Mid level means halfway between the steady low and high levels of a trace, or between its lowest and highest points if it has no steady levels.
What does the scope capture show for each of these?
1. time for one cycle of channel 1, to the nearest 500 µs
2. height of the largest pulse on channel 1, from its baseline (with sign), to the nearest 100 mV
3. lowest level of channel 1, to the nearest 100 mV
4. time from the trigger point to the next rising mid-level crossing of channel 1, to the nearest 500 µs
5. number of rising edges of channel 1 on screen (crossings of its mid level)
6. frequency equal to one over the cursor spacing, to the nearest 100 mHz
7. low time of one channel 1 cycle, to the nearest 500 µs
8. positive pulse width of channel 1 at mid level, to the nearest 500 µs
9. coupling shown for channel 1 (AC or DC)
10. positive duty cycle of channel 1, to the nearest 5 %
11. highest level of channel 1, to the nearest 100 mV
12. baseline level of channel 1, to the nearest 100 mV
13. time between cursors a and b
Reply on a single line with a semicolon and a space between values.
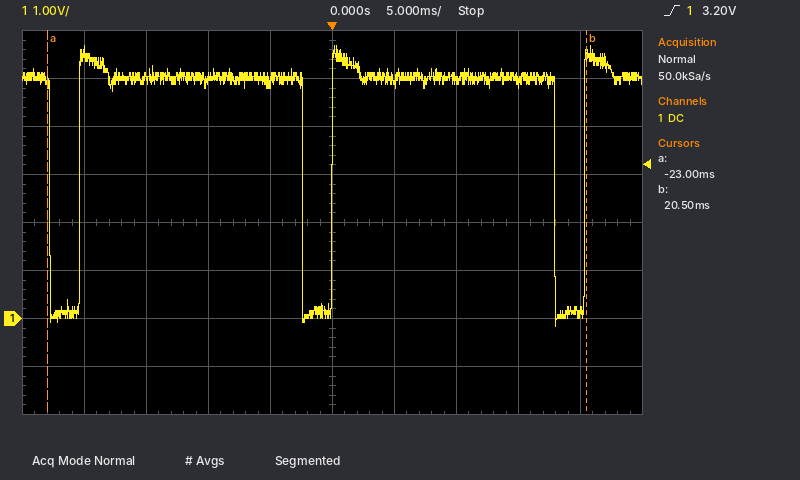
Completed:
20.5 ms; -5.2 V; -200 mV; 20.5 ms; 3; 23.0 Hz; 2.5 ms; 18.0 ms; DC; 90 %; 5.7 V; 5.0 V; 43.5 ms
